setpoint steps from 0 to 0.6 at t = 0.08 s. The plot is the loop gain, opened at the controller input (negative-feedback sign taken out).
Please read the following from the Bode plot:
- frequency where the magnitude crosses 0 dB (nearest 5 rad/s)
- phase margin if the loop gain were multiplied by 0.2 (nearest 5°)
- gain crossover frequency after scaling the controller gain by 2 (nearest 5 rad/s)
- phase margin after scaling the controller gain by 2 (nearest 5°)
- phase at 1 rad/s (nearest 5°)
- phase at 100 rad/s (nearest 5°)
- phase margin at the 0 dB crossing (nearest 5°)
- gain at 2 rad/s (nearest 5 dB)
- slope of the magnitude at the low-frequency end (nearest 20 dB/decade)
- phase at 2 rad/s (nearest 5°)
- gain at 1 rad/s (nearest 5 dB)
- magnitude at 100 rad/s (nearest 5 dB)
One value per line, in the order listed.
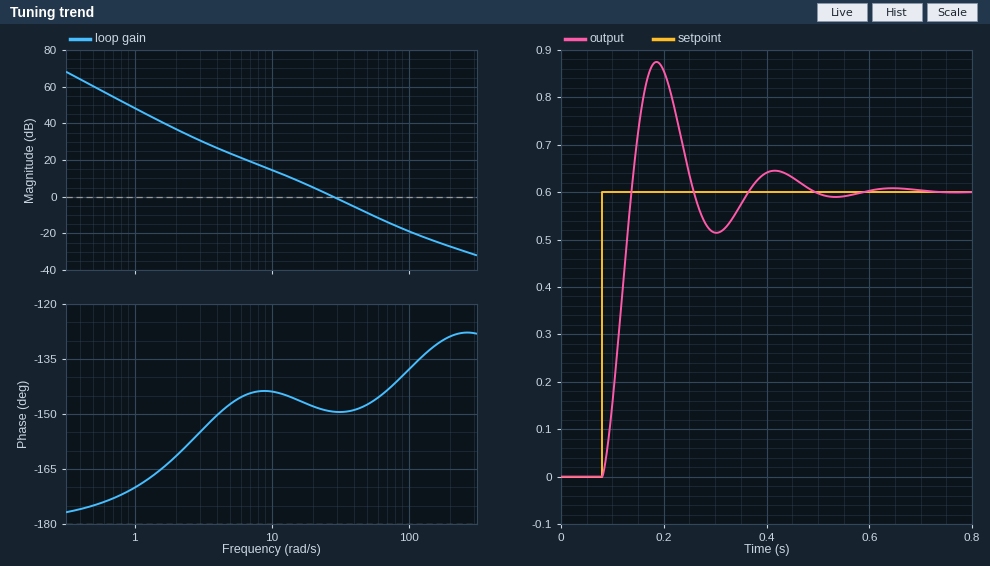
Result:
30 rad/s
35°
40 rad/s
30°
-170°
-140°
30°
35 dB
-40 dB/decade
-160°
50 dB
-20 dB
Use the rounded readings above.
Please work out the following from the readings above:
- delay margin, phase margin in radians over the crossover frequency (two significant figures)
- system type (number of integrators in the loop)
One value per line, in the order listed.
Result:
0.017 s
2
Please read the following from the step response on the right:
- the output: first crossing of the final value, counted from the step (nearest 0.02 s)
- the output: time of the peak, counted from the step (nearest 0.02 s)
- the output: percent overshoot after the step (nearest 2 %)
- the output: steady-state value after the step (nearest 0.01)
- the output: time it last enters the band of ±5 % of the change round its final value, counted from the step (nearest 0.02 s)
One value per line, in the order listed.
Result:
0.06 s
0.10 s
46 %
0.60
0.38 s
